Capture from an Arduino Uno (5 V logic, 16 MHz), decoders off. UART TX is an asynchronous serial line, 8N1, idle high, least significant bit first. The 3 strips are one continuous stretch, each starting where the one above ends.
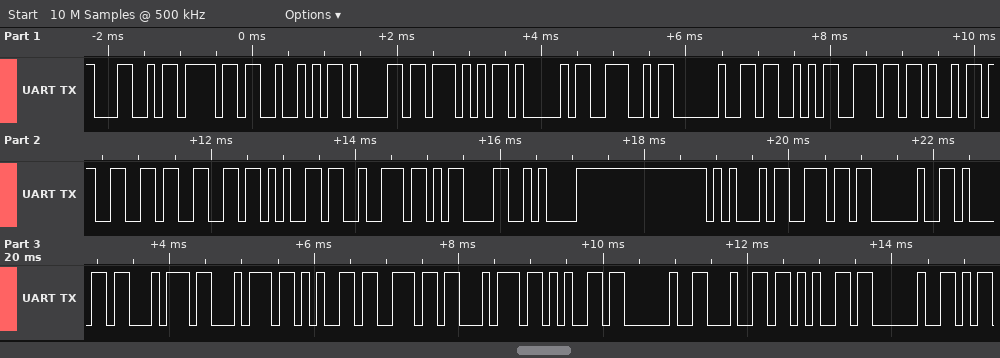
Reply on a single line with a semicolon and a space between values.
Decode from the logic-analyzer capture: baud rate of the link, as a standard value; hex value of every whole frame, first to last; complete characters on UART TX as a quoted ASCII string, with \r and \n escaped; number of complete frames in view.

9600 baud; 4C 6F 52 61 57 41 4E 20 53 6E 69 66 66 65 72 0D 0A 45 6E 20 61 74 74 65 6E 74 65 20 64 65 20; "LoRaWAN Sniffer\r\nEn attente de "; 31
